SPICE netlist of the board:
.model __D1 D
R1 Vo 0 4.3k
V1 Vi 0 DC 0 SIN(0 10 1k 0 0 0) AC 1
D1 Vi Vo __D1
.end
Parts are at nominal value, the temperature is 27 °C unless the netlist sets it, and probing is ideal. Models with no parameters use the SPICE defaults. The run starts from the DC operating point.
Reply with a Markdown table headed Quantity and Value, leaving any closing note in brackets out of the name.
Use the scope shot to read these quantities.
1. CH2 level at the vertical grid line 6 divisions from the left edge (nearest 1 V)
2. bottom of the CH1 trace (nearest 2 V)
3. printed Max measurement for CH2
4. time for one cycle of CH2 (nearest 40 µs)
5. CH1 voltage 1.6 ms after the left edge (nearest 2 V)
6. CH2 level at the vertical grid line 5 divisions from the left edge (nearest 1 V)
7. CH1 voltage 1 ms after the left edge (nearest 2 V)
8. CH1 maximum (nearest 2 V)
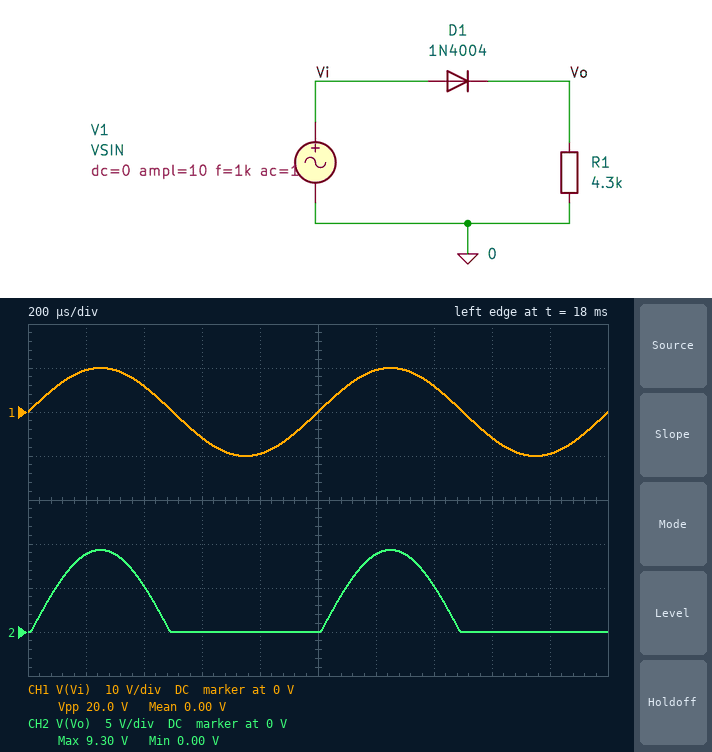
| Quantity | Value |
|---|---|
| CH2 level at the vertical grid line 6 divisions from the left edge | 9 V |
| bottom of the CH1 trace | -10 V |
| printed Max measurement for CH2 | 9.30 V |
| time for one cycle of CH2 | 1.00 ms |
| CH1 voltage 1.6 ms after the left edge | -6 V |
| CH2 level at the vertical grid line 5 divisions from the left edge | 0 V |
| CH1 voltage 1 ms after the left edge | 0 V |
| CH1 maximum | 10 V |
